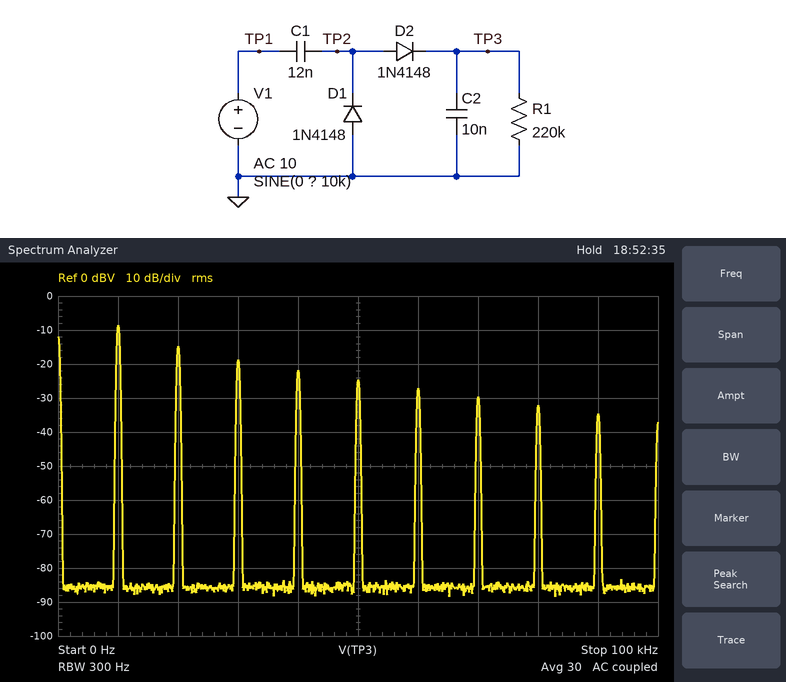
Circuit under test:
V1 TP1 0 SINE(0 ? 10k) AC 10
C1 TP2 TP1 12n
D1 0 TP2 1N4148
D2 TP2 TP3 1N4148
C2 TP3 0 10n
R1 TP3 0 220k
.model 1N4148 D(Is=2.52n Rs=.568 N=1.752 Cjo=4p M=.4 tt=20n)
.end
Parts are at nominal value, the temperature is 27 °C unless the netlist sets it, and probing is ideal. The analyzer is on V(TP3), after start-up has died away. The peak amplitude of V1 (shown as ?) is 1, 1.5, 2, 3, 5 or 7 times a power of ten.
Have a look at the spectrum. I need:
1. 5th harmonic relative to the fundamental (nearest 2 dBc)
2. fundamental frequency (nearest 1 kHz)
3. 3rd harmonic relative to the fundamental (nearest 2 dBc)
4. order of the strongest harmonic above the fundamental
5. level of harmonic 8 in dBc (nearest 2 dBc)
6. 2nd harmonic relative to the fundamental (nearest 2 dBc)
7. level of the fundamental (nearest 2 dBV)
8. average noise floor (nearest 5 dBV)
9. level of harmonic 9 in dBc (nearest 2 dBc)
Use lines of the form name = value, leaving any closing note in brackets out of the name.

5th harmonic relative to the fundamental = -16 dBc
fundamental frequency = 10 kHz
3rd harmonic relative to the fundamental = -10 dBc
order of the strongest harmonic above the fundamental = 2
level of harmonic 8 in dBc = -24 dBc
2nd harmonic relative to the fundamental = -6 dBc
level of the fundamental = -8 dBV
average noise floor = -85 dBV
level of harmonic 9 in dBc = -26 dBc
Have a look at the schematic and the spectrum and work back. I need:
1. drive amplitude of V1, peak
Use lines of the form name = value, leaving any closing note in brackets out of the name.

drive amplitude of V1, peak = 20 V
